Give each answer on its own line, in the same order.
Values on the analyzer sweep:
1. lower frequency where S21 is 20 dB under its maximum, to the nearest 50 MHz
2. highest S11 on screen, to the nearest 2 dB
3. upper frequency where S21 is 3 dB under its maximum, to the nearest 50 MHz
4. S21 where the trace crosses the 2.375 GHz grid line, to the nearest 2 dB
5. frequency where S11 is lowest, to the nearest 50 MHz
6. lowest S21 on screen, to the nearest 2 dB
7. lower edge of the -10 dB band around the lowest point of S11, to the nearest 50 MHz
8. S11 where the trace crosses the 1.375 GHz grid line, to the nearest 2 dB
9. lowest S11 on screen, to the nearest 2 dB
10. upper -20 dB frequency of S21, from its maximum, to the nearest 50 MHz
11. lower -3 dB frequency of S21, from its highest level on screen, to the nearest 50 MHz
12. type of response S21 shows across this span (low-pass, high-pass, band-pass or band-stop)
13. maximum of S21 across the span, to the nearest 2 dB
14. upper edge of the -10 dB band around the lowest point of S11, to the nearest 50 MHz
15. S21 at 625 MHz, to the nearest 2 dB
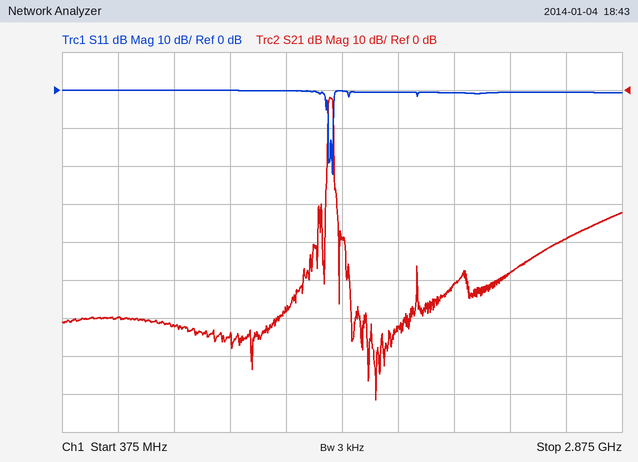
1.55 GHz
0 dB
1.60 GHz
-48 dB
1.60 GHz
-82 dB
1.55 GHz
0 dB
-22 dB
1.60 GHz
1.55 GHz
band-pass
-2 dB
1.60 GHz
-60 dB
